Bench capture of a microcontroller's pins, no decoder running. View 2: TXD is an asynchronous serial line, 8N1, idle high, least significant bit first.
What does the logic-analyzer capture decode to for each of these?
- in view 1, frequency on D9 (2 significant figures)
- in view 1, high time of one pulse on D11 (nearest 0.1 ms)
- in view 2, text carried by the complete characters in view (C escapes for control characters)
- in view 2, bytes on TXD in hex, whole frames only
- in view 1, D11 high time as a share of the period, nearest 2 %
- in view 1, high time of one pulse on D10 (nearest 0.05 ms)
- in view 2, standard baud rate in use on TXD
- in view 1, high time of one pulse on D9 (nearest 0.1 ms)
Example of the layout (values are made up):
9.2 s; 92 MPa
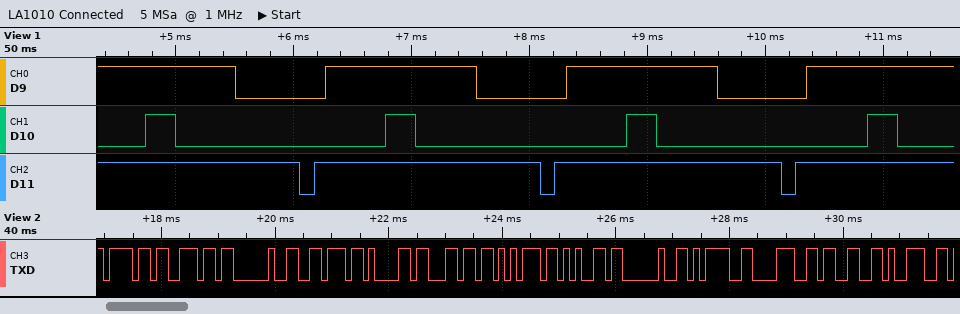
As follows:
490 Hz; 1.9 ms; "on value =839"; 6F 6E 20 76 61 6C 75 65 20 3D 38 33 39; 94 %; 0.25 ms; 9600 baud; 1.3 ms
